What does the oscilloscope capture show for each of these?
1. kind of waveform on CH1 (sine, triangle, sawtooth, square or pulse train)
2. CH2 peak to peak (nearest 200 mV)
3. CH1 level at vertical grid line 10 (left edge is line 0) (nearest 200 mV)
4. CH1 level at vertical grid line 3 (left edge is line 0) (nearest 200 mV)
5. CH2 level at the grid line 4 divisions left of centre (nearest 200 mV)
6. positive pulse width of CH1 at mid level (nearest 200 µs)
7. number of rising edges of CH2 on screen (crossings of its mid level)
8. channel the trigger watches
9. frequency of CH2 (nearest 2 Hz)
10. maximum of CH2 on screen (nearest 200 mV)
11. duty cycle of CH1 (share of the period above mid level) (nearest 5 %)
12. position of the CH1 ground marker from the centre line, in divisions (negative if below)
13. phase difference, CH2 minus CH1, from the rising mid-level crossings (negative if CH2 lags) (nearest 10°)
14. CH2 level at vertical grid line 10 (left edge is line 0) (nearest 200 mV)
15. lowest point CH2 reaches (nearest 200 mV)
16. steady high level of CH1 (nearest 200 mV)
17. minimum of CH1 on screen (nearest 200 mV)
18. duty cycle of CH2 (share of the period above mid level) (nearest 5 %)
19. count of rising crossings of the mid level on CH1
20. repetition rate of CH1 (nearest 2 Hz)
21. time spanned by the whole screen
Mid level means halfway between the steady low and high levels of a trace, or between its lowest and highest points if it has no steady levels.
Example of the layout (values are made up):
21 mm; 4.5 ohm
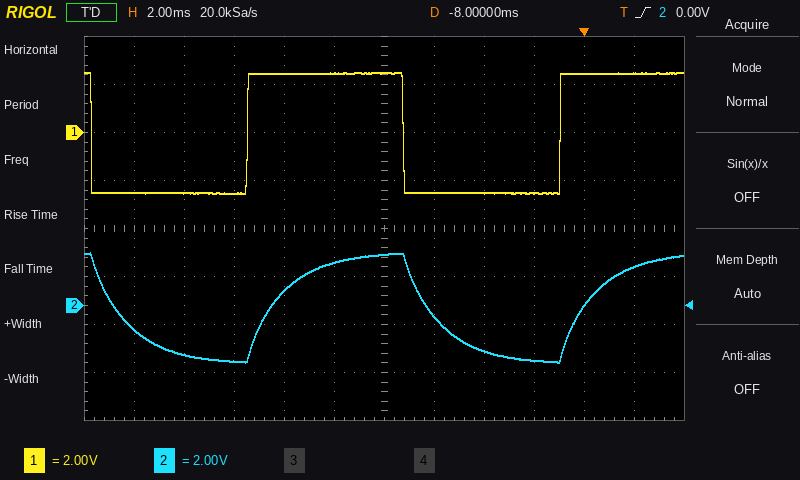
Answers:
square; 4.6 V; 2.4 V; -2.6 V; -2.0 V; 6.2 ms; 2; CH2; 80 Hz; 2.2 V; 50 %; +2.0 div; -30°; 0.0 V; -2.4 V; 2.4 V; -2.6 V; 50 %; 2; 80 Hz; 24 ms
